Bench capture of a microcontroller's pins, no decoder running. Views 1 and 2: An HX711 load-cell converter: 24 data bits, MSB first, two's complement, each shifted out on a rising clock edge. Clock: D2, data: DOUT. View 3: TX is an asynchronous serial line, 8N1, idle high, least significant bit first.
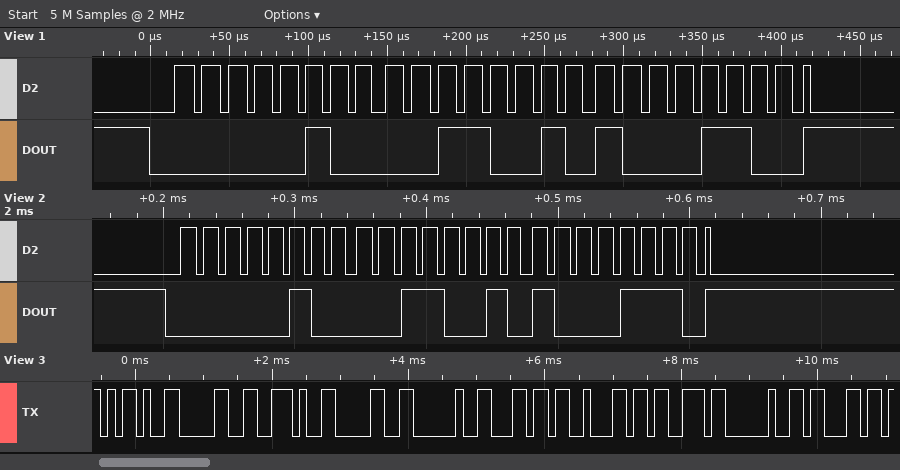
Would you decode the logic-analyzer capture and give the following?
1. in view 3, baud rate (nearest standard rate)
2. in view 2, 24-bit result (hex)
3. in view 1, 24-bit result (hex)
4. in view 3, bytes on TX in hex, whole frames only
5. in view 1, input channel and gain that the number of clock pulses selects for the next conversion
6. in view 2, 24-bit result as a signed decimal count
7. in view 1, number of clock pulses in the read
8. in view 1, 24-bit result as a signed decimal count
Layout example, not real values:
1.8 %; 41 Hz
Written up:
9600 baud; 0x04328E; 0x04328C; 2D 30 2E 30 20 6C 62 73 20 63; channel A, gain 128; 275086; 25; 275084
